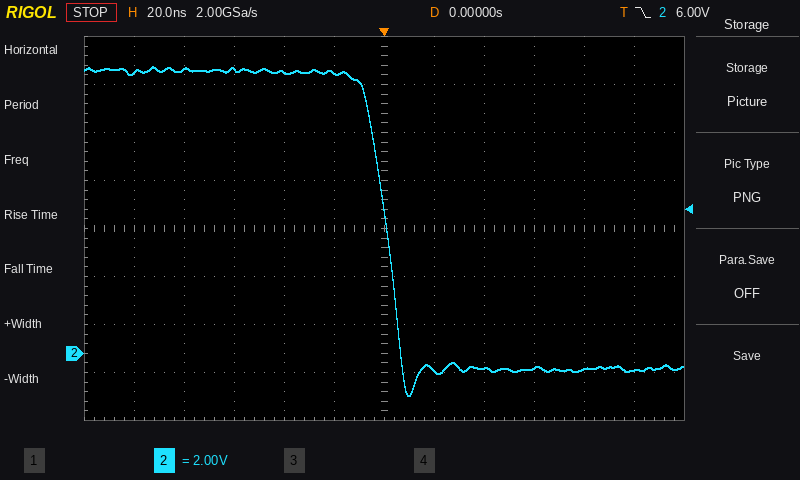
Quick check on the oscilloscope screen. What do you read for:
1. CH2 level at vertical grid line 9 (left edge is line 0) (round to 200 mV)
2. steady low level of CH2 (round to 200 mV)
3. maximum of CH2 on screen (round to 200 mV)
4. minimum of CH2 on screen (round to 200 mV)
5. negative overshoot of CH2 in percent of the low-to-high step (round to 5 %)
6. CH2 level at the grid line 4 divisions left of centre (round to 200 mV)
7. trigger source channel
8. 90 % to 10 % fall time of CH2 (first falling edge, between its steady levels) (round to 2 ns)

-600 mV
-600 mV
12.0 V
-1.8 V
10 %
11.8 V
CH2
14 ns
